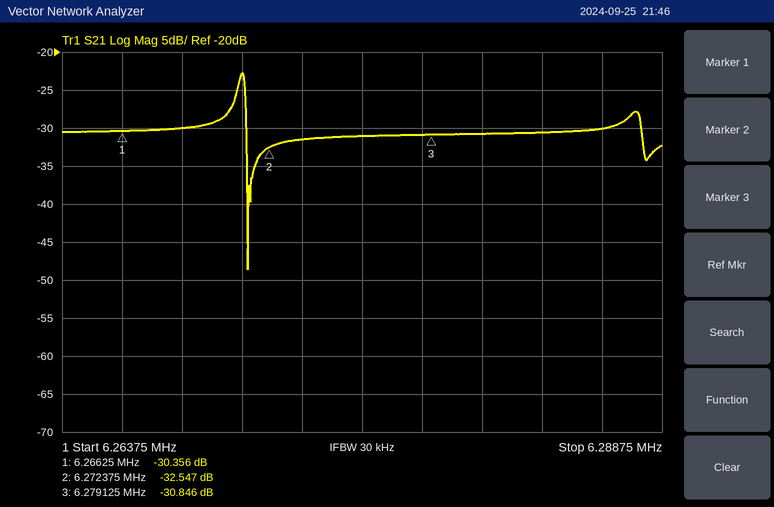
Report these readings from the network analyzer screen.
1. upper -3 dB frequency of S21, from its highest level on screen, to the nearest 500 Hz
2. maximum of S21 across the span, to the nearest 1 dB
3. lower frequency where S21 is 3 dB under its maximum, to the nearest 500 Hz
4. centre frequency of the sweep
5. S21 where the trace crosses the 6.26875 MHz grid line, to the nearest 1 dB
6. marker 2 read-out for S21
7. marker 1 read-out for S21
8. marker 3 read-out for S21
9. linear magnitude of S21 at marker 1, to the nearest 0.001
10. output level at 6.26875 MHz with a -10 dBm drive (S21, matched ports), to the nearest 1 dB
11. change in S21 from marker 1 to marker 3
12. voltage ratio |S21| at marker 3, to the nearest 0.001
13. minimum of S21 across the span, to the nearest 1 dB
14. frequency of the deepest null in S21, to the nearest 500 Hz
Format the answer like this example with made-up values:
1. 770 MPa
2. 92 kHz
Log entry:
1. 6.2715 MHz
2. -23 dB
3. 6.2710 MHz
4. 6.27625 MHz
5. -30 dB
6. -32.547 dB
7. -30.356 dB
8. -30.846 dB
9. 0.030
10. -40 dBm
11. -0.490 dB
12. 0.029
13. -49 dB
14. 6.2715 MHz
